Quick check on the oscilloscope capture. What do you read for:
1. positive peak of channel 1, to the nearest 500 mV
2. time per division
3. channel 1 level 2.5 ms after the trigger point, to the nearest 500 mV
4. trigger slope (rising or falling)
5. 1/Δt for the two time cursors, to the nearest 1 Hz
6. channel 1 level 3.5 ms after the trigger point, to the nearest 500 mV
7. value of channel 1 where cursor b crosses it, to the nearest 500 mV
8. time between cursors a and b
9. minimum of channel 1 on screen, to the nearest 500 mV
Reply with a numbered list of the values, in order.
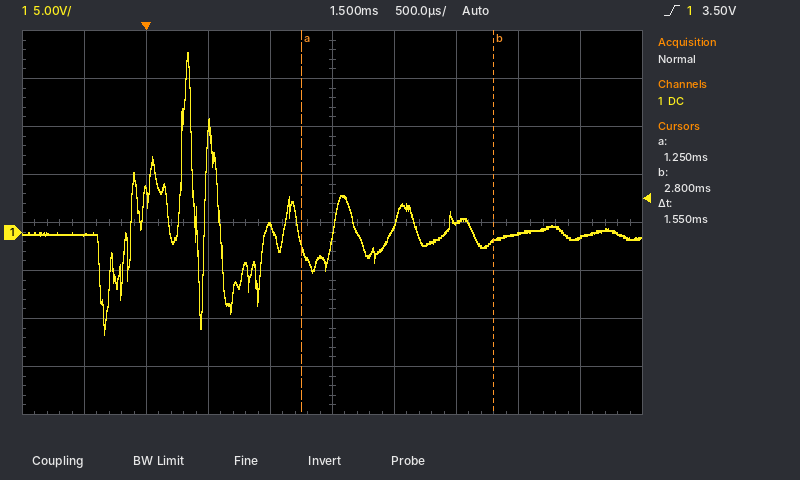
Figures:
1. 18.5 V
2. 500 µs
3. 1.0 V
4. rising
5. 645 Hz
6. -500 mV
7. -1.0 V
8. 1.55 ms
9. -10.5 V
